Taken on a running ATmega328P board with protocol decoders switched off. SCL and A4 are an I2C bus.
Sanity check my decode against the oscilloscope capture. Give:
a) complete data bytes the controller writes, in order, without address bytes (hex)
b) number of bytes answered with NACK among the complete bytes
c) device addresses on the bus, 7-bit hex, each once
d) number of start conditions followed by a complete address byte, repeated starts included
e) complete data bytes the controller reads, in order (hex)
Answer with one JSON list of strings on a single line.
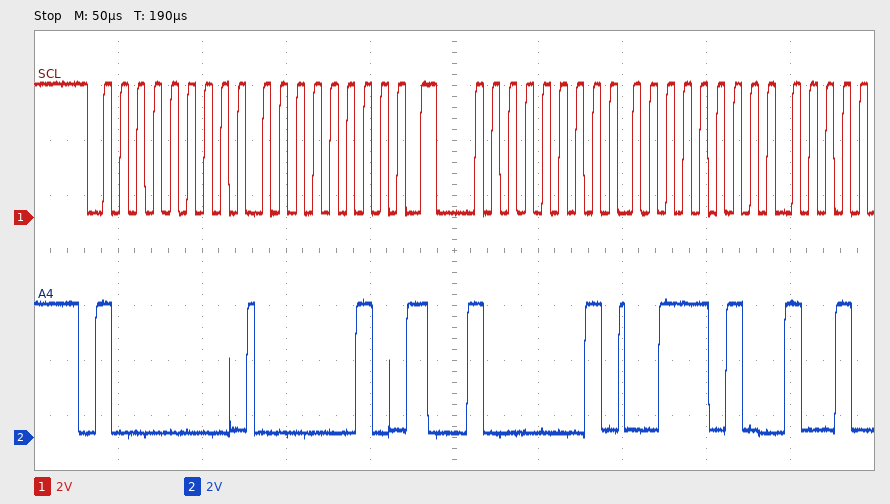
["02", "0", "0x40", "2", "3A"]
